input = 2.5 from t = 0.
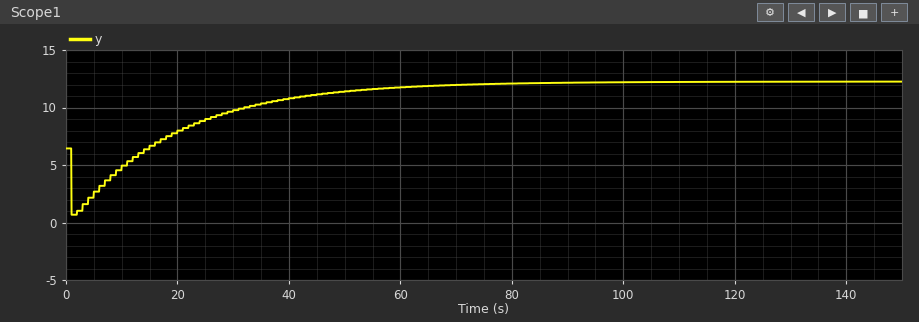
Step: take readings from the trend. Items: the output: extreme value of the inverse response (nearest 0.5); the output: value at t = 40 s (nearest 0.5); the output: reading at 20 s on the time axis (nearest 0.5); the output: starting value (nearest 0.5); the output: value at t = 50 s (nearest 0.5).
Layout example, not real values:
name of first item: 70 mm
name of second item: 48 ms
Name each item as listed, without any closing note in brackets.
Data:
the output: extreme value of the inverse response: 0.5
the output: value at t = 40 s: 11.0
the output: reading at 20 s on the time axis: 8.0
the output: starting value: 6.5
the output: value at t = 50 s: 11.5
